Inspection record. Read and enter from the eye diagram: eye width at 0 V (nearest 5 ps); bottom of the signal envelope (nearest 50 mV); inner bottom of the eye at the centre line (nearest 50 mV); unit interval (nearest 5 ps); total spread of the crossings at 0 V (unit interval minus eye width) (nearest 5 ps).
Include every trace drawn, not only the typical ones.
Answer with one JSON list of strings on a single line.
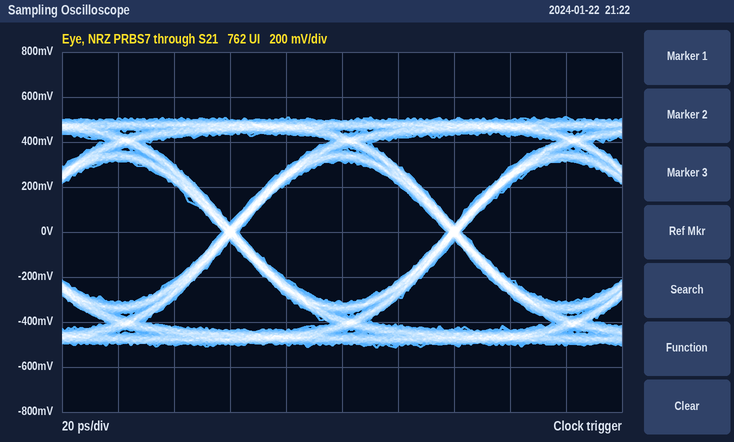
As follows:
["75 ps", "-500 mV", "-300 mV", "80 ps", "5 ps"]
